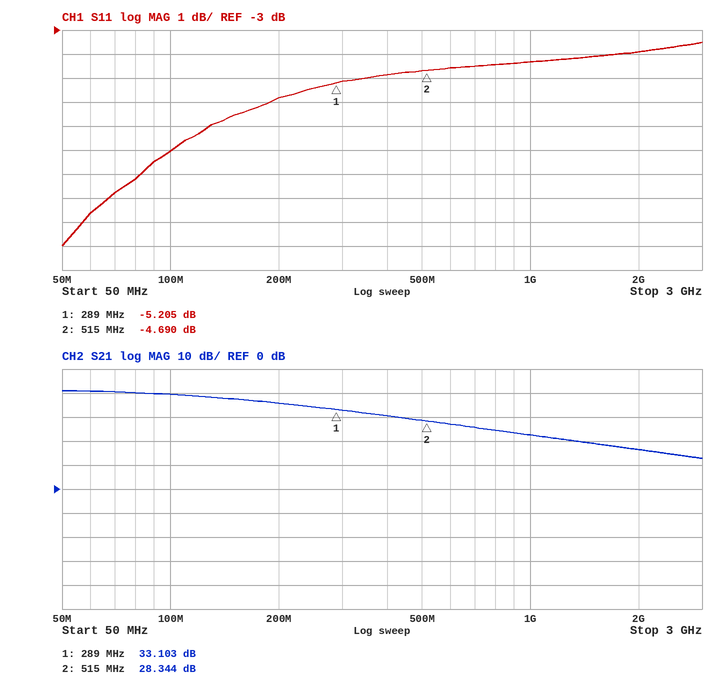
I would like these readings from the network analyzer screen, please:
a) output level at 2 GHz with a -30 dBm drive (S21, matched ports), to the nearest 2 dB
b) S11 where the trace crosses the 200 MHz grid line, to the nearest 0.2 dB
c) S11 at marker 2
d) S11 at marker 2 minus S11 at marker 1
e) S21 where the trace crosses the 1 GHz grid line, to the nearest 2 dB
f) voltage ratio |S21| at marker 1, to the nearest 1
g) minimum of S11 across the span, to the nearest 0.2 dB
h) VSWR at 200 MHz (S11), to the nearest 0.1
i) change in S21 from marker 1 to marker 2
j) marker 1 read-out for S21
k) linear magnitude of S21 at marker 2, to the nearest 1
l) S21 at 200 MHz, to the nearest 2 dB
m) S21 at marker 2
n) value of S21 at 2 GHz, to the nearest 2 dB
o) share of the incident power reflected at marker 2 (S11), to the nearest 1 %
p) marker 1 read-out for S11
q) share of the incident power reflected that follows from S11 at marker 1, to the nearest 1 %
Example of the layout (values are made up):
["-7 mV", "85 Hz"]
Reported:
["-14 dBm", "-5.8 dB", "-4.690 dB", "0.515 dB", "22 dB", "45", "-12.0 dB", "3.1", "-4.759 dB", "33.103 dB", "26", "36 dB", "28.344 dB", "16 dB", "34 %", "-5.205 dB", "30 %"]
